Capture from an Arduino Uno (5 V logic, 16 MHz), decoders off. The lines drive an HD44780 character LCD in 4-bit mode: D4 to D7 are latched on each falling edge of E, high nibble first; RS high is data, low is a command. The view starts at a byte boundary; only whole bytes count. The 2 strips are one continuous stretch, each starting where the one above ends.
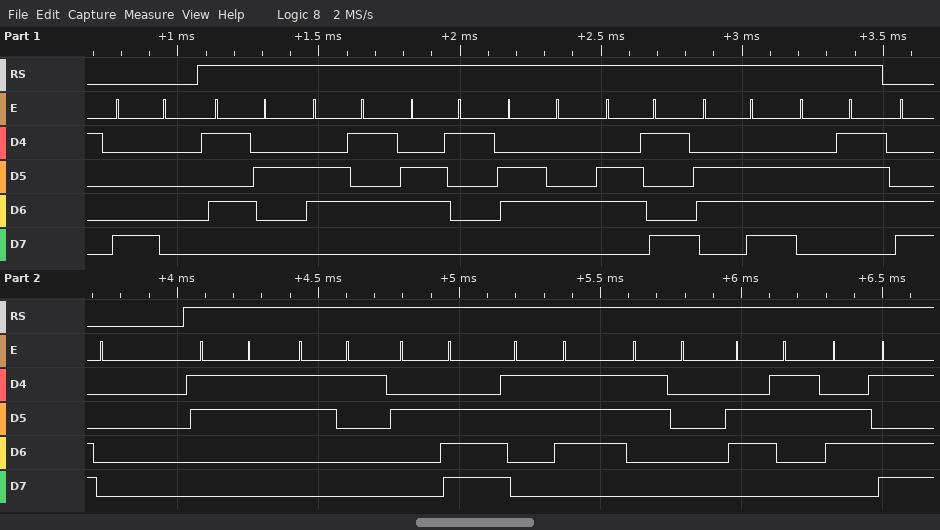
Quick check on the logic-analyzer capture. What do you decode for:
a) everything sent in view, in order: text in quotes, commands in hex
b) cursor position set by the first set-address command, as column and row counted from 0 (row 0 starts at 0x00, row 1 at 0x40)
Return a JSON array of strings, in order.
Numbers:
["0x80 \"Reading\" 0xC0 \"31.70cm\"", "column 0, row 0"]
